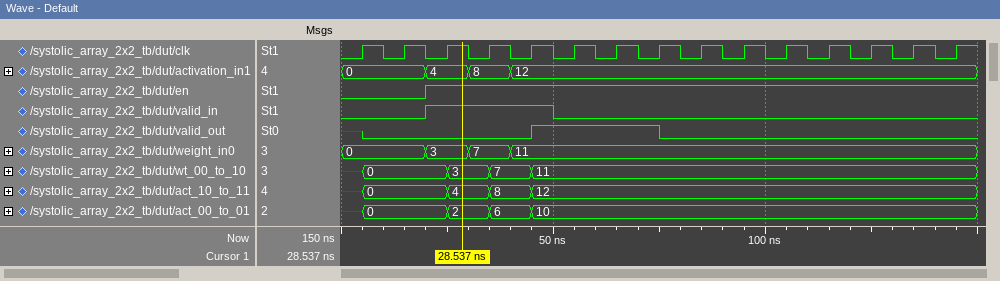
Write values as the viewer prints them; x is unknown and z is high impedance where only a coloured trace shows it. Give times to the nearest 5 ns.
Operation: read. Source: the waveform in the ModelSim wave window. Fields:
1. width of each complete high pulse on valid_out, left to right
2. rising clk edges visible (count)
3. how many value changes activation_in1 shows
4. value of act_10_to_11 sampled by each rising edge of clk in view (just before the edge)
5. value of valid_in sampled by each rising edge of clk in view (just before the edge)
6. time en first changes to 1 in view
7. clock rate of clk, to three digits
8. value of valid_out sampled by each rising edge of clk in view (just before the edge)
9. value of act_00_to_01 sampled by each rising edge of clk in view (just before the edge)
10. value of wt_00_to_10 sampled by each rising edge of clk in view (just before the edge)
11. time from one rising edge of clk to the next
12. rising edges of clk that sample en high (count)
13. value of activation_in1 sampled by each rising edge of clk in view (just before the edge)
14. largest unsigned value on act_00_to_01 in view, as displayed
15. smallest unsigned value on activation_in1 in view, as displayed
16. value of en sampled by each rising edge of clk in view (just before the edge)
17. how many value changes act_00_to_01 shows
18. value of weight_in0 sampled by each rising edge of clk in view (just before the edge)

30 ns
15
3
x, 0, 0, 4, 8, 12, 12, 12, 12, 12, 12, 12, 12, 12, 12
0 0 1 1 1 0 0 0 0 0 0 0 0 0 0
20 ns
100 MHz
x 0 0 0 0 1 1 1 0 0 0 0 0 0 0
x, 0, 0, 2, 6, 10, 10, 10, 10, 10, 10, 10, 10, 10, 10
x, 0, 0, 3, 7, 11, 11, 11, 11, 11, 11, 11, 11, 11, 11
10 ns
13
0, 0, 4, 8, 12, 12, 12, 12, 12, 12, 12, 12, 12, 12, 12
10
0
0 0 1 1 1 1 1 1 1 1 1 1 1 1 1
4
0, 0, 3, 7, 11, 11, 11, 11, 11, 11, 11, 11, 11, 11, 11
